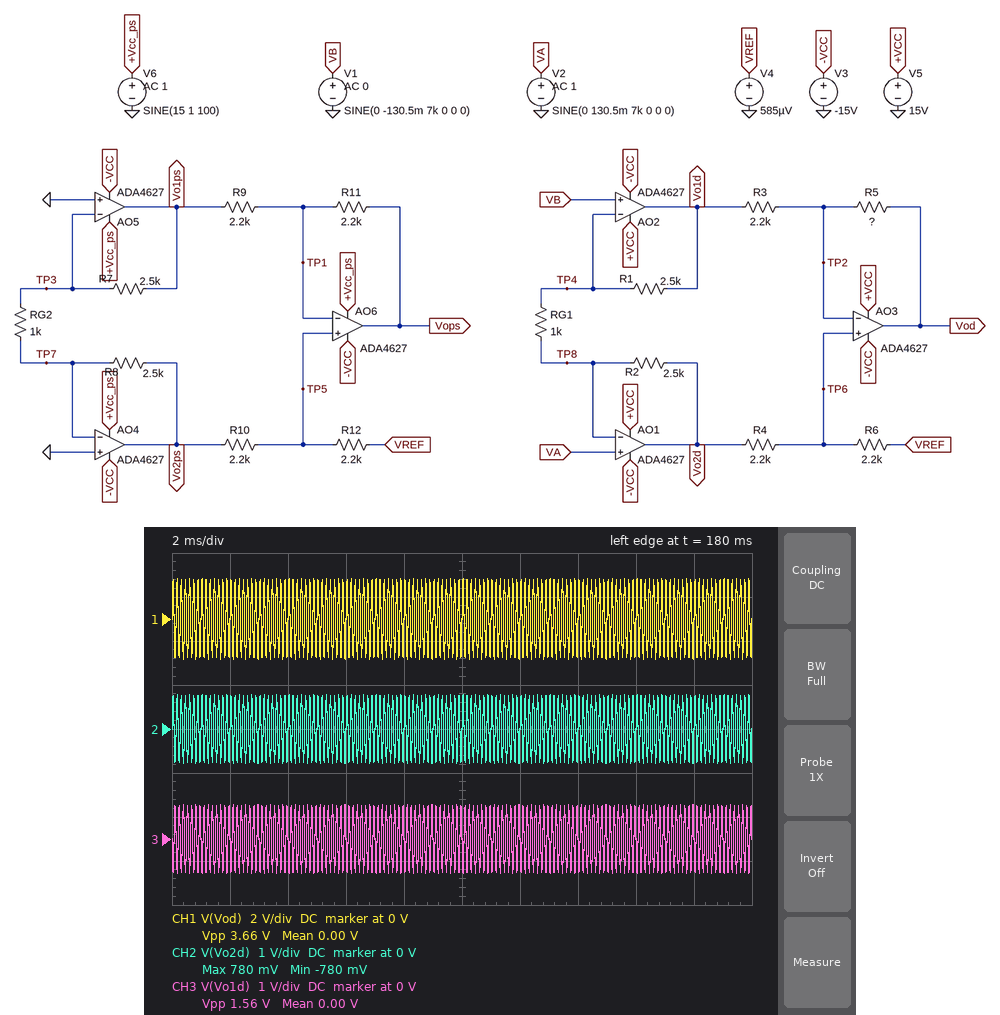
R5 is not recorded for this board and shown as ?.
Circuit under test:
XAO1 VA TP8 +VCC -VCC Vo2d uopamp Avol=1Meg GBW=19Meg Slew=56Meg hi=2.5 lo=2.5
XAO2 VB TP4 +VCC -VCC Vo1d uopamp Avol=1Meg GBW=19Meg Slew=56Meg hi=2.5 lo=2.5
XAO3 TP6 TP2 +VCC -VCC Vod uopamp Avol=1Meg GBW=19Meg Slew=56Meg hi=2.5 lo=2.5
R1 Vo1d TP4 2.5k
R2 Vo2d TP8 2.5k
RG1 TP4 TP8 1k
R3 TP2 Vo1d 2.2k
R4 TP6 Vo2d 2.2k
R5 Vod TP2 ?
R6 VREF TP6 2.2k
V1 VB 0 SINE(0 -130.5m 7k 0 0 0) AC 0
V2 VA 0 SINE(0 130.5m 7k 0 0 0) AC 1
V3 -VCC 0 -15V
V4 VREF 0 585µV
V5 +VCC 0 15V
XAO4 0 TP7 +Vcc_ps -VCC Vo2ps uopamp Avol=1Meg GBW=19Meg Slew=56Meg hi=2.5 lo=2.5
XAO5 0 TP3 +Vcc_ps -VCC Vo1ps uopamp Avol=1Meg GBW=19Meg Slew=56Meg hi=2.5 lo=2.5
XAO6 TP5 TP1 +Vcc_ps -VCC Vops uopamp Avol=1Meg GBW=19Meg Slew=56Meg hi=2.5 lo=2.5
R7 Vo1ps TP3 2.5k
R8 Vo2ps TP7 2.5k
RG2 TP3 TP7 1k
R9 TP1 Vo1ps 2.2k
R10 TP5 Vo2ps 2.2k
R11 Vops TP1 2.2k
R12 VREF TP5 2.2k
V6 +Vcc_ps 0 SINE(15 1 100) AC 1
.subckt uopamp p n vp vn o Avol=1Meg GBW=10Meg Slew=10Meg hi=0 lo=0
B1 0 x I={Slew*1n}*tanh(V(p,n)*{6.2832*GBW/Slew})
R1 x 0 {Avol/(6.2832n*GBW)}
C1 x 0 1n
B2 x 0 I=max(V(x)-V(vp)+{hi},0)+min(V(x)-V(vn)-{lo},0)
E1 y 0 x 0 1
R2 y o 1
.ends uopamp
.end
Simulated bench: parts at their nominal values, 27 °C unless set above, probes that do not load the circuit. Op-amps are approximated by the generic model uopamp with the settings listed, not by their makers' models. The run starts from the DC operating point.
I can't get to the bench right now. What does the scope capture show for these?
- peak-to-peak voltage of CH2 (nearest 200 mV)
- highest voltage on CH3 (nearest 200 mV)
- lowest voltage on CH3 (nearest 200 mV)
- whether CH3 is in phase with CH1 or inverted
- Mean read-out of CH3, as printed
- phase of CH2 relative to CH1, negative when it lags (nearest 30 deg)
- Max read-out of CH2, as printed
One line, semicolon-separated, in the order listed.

1.6 V; 800 mV; -800 mV; inverted; 0.00 V; 0 deg; 780 mV
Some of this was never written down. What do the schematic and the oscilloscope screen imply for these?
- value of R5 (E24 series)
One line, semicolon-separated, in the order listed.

2.7 kΩ
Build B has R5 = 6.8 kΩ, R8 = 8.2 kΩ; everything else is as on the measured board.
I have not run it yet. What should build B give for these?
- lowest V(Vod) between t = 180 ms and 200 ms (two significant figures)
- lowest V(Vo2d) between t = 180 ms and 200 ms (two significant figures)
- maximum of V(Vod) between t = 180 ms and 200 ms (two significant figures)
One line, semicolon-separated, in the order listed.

-4.0 V; -780 mV; 4.0 V
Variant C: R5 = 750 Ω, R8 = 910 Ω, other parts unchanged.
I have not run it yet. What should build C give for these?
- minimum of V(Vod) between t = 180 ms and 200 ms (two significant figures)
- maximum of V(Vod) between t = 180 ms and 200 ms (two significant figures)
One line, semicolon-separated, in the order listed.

-790 mV; 790 mV
